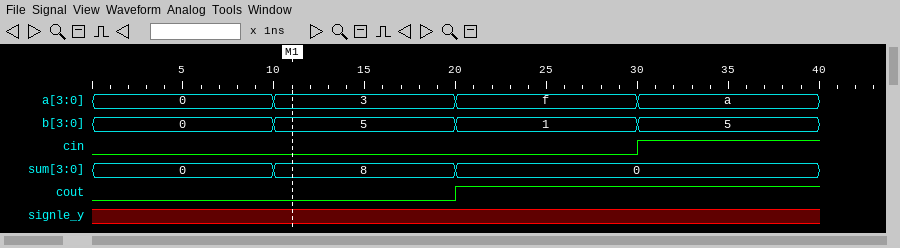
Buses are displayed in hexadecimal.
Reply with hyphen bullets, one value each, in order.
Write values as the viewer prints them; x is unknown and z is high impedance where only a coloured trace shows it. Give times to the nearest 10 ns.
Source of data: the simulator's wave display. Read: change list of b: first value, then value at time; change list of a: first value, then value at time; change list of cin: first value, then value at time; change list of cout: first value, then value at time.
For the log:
- 0, 5 at 10 ns, 1 at 20 ns, 5 at 30 ns
- 0, 3 at 10 ns, f at 20 ns, a at 30 ns
- 0, 1 at 30 ns
- 0, 1 at 20 ns
